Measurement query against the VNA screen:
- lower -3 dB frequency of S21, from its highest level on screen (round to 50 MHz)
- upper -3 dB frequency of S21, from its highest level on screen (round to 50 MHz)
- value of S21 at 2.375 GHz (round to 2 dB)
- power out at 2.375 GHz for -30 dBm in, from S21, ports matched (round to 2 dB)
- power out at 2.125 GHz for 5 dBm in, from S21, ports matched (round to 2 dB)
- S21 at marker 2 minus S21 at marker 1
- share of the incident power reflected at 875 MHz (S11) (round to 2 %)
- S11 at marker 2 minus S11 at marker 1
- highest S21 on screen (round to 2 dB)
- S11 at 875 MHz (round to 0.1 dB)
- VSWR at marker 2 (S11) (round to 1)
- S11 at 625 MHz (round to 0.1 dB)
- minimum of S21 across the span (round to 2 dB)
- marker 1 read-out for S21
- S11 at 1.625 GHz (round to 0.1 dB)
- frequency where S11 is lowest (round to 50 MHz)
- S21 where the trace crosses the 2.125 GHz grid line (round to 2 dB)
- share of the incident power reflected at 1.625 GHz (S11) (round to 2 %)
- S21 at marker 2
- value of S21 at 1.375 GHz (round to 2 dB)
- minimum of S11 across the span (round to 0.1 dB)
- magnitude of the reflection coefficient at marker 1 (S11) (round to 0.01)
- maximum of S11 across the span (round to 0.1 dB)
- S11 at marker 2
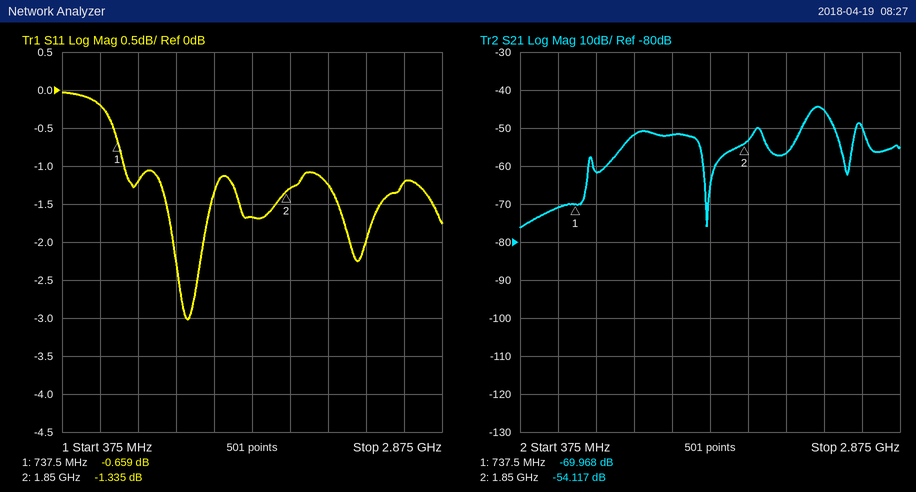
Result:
2.25 GHz
2.40 GHz
-46 dB
-76 dBm
-52 dBm
15.851 dB
76 %
-0.676 dB
-44 dB
-1.2 dB
13
-0.2 dB
-76 dB
-69.968 dB
-1.7 dB
1.20 GHz
-56 dB
68 %
-54.117 dB
-52 dB
-3.0 dB
0.93
0.0 dB
-1.335 dB
